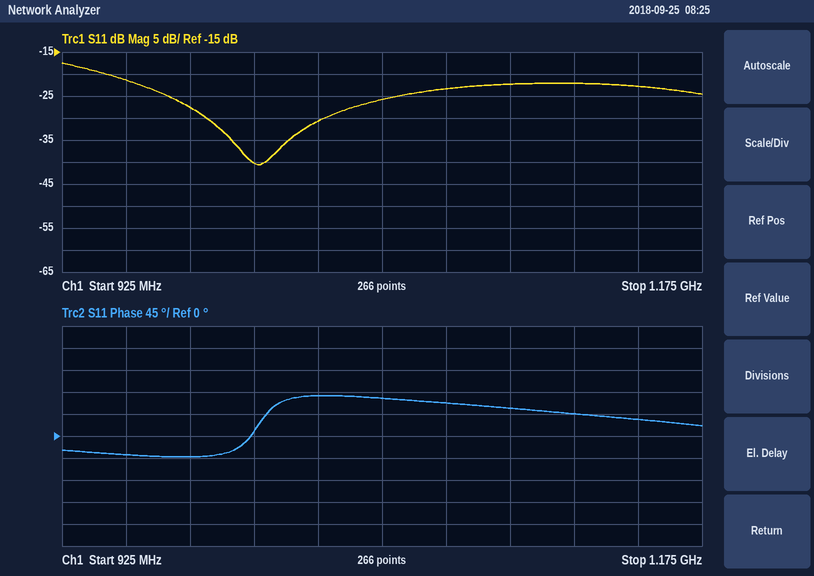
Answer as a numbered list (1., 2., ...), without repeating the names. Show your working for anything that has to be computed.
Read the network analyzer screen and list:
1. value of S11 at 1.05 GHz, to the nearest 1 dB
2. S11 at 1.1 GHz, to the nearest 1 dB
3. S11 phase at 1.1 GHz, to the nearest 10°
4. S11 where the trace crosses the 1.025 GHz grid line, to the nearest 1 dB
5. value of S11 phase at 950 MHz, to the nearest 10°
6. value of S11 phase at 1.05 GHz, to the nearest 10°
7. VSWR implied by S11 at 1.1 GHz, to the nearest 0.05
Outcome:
1. -26 dB
2. -22 dB
3. 60°
4. -31 dB
5. -40°
6. 80°
7. |Γ| = 10^(-22/20) = 0.0794; VSWR = (1 + 0.0794)/(1 − 0.0794) ≈ 1.17, so 1.15 to the nearest 0.05
